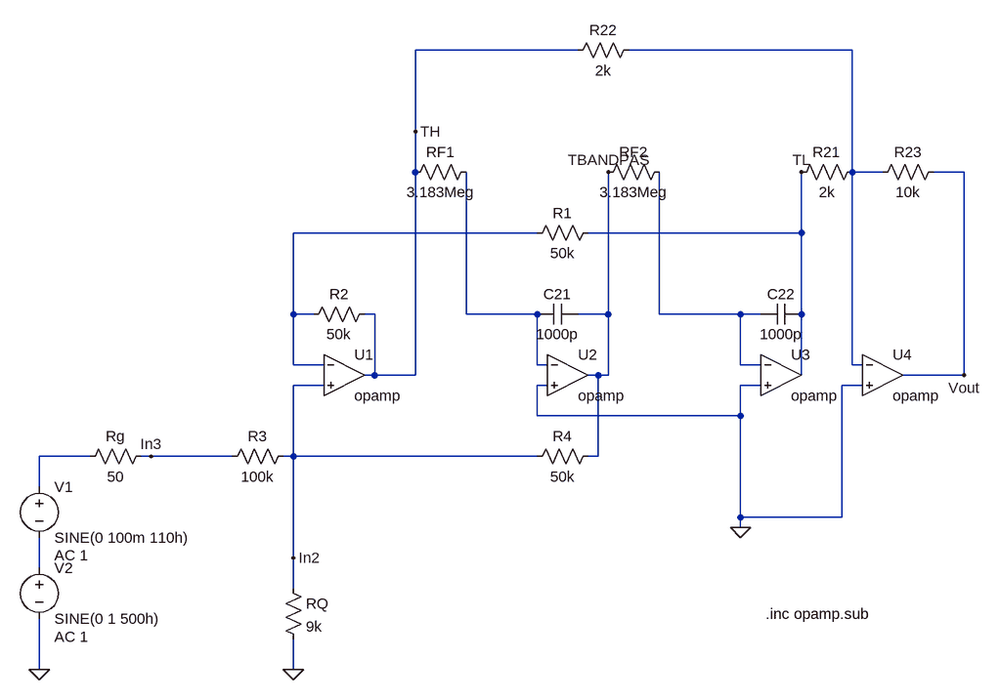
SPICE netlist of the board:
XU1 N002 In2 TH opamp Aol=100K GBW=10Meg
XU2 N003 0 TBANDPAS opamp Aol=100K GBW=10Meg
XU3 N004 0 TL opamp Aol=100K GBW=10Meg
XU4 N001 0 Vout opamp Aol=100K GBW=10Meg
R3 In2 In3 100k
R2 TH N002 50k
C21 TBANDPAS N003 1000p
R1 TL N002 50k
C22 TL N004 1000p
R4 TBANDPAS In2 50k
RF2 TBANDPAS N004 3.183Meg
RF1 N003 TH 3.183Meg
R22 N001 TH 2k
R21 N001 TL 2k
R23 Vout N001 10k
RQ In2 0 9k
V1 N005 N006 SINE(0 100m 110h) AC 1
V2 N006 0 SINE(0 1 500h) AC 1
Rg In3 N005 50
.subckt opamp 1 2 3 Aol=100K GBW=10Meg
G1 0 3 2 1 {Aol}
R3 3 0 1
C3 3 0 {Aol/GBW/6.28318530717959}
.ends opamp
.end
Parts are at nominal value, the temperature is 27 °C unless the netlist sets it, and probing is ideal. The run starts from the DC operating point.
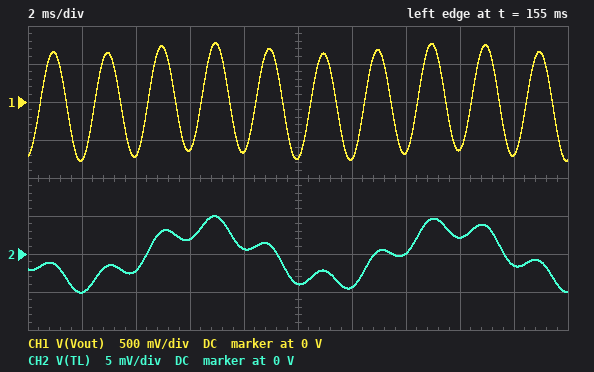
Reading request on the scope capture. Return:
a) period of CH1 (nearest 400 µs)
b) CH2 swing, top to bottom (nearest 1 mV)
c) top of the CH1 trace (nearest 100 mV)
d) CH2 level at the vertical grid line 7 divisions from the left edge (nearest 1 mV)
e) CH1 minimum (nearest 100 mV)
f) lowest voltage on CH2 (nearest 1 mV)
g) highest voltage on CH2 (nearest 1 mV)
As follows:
2.0 ms
10 mV
800 mV
0 V
-800 mV
-5 mV
5 mV
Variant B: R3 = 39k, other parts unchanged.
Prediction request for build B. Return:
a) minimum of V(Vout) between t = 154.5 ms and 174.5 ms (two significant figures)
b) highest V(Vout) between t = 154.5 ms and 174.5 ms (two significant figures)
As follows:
-1.8 V
1.8 V
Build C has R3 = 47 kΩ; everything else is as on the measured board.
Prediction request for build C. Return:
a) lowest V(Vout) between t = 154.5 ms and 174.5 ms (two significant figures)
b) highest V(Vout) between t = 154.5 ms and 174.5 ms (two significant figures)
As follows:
-1.5 V
1.5 V
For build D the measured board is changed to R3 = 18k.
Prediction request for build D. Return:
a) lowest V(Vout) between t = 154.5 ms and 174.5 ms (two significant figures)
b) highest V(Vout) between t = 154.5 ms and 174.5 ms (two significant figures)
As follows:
-3.3 V
3.3 V
